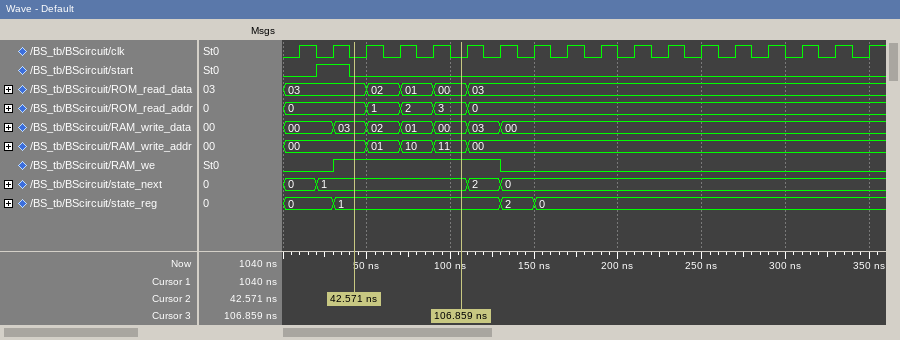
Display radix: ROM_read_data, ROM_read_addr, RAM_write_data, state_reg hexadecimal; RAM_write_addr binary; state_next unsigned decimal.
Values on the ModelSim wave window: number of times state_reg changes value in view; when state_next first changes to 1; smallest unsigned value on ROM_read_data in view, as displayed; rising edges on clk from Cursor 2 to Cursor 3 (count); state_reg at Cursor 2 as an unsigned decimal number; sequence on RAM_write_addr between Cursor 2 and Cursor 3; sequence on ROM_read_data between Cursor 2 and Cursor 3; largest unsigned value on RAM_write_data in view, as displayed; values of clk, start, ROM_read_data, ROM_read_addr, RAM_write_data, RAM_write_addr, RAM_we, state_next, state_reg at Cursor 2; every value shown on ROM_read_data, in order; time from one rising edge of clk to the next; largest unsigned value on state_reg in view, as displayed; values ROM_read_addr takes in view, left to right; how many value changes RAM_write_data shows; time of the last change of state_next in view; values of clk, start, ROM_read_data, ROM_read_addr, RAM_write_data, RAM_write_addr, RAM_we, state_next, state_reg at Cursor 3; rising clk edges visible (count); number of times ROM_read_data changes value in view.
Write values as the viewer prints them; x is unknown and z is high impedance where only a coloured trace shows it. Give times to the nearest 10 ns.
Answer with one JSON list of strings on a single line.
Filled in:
["3", "20 ns", "00", "3", "1", "00, 01, 10, 11", "03, 02, 01, 00", "03", "clk=0, start=0, ROM_read_data=03, ROM_read_addr=0, RAM_write_data=03, RAM_write_addr=00, RAM_we=1, state_next=1, state_reg=1", "03, 02, 01, 00, 03", "20 ns", "2", "0, 1, 2, 3, 0", "6", "130 ns", "clk=0, start=0, ROM_read_data=00, ROM_read_addr=3, RAM_write_data=00, RAM_write_addr=11, RAM_we=1, state_next=1, state_reg=1", "18", "4"]
